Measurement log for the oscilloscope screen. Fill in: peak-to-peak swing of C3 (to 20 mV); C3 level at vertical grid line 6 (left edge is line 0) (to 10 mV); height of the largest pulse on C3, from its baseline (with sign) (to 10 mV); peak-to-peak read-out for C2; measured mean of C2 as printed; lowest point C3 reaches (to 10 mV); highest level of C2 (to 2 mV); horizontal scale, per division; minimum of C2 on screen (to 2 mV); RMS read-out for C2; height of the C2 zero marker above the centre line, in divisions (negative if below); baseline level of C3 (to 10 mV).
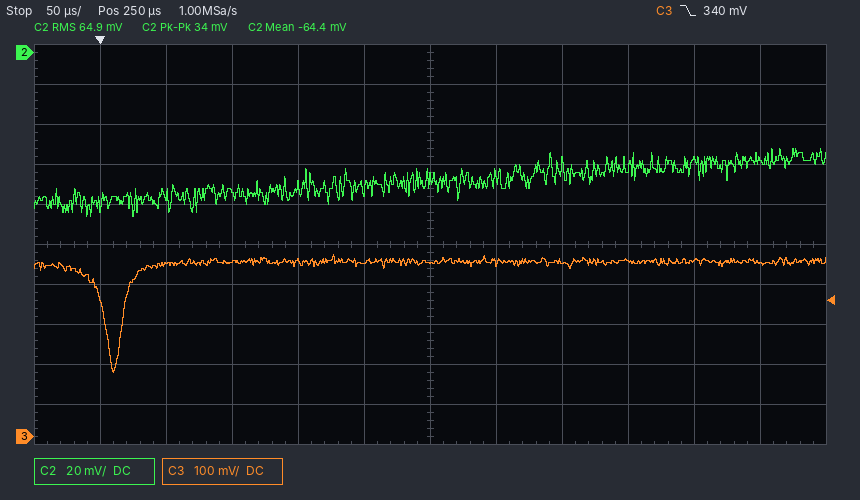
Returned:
300 mV
430 mV
-280 mV
34 mV
-64.4 mV
160 mV
-48 mV
50 µs
-82 mV
64.9 mV
+4.8 div
440 mV
